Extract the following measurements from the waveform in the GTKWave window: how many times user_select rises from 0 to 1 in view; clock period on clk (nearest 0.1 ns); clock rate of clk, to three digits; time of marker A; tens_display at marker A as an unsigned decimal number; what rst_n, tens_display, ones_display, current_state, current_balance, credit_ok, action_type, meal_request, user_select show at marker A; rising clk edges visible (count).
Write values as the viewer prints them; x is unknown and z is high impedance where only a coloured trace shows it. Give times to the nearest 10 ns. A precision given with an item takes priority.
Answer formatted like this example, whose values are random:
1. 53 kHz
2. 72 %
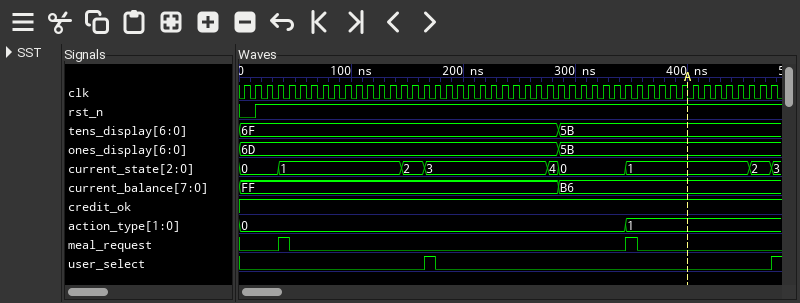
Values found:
1. 2
2. 10 ns
3. 100 MHz
4. 400 ns
5. 91
6. rst_n=1, tens_display=5B, ones_display=5B, current_state=1, current_balance=B6, credit_ok=1, action_type=1, meal_request=0, user_select=0
7. 48
